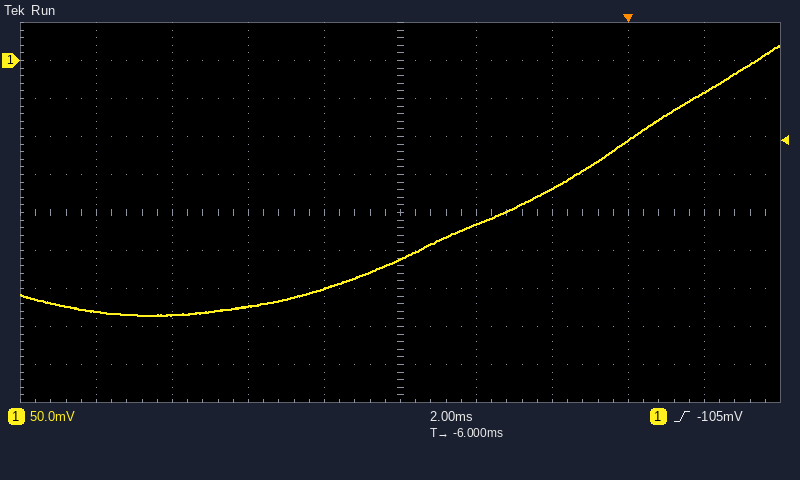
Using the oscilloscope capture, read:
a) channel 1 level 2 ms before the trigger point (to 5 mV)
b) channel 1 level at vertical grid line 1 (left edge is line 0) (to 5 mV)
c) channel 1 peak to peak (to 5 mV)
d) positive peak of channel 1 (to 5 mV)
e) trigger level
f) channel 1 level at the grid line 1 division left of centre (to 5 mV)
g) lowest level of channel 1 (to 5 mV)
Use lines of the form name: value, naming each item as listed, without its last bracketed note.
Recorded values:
channel 1 level 2 ms before the trigger point: -170 mV
channel 1 level at vertical grid line 1 (left edge is line 0): -330 mV
channel 1 peak to peak: 355 mV
positive peak of channel 1: 20 mV
trigger level: -105 mV
channel 1 level at the grid line 1 division left of centre: -300 mV
lowest level of channel 1: -335 mV
